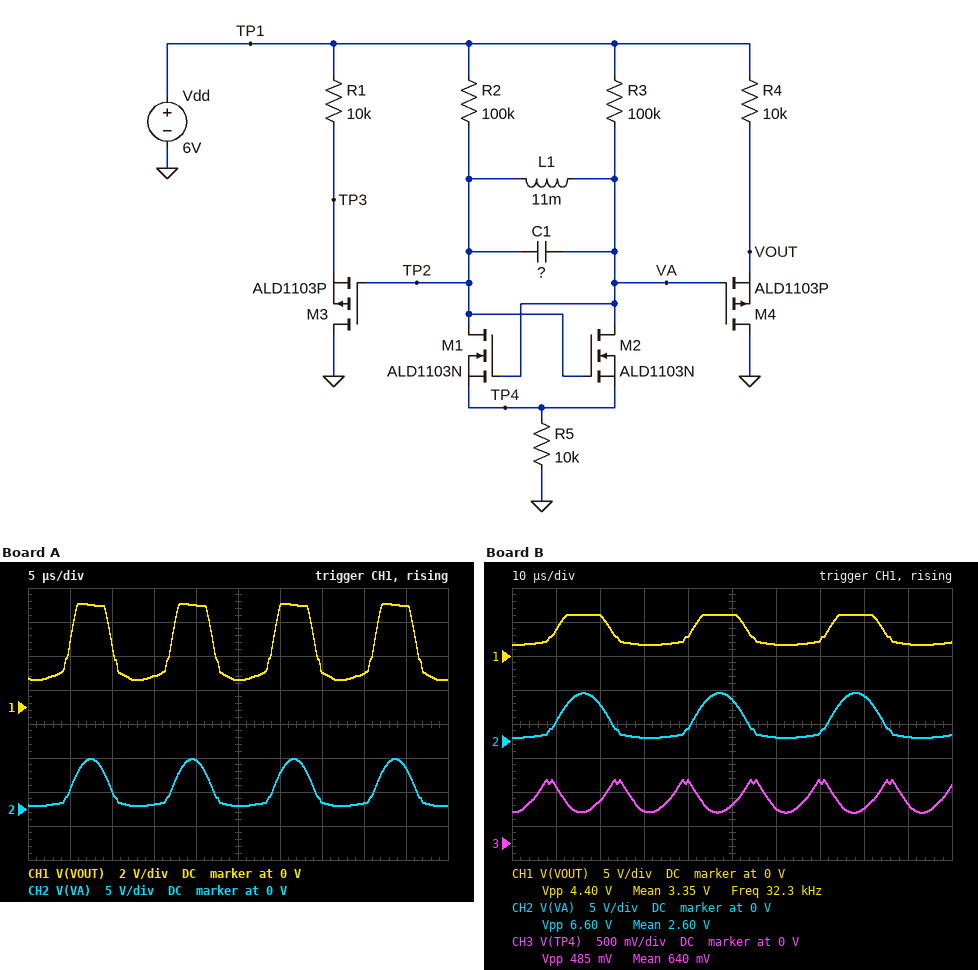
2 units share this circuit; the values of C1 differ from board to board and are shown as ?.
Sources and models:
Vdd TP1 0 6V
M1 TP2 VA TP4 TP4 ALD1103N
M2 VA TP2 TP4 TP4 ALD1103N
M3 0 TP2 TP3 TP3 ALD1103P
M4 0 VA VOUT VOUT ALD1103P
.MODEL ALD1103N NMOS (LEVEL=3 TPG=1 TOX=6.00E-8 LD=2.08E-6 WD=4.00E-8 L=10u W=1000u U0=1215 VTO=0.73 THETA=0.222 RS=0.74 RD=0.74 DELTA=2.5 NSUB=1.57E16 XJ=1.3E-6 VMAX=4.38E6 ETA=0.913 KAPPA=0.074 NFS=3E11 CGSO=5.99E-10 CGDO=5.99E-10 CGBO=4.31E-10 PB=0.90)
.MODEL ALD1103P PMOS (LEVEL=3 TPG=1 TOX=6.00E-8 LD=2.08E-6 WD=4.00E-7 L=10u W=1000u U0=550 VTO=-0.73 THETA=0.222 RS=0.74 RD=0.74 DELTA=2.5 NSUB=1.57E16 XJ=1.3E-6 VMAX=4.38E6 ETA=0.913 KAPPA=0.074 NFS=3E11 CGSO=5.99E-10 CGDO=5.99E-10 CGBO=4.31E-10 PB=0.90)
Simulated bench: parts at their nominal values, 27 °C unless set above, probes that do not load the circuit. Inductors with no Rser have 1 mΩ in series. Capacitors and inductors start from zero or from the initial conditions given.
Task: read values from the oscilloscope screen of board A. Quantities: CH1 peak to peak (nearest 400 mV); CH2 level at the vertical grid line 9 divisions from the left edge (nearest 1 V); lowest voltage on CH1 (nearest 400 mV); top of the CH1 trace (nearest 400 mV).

4.4 V
6 V
1.6 V
6.0 V
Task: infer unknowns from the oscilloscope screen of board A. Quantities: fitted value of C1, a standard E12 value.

330 pF
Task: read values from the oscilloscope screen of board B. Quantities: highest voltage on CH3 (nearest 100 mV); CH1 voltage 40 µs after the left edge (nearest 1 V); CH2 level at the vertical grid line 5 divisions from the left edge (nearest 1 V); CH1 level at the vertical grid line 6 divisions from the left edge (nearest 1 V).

900 mV
3 V
6 V
2 V
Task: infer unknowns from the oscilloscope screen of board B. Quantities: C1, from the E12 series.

2.2 nF
